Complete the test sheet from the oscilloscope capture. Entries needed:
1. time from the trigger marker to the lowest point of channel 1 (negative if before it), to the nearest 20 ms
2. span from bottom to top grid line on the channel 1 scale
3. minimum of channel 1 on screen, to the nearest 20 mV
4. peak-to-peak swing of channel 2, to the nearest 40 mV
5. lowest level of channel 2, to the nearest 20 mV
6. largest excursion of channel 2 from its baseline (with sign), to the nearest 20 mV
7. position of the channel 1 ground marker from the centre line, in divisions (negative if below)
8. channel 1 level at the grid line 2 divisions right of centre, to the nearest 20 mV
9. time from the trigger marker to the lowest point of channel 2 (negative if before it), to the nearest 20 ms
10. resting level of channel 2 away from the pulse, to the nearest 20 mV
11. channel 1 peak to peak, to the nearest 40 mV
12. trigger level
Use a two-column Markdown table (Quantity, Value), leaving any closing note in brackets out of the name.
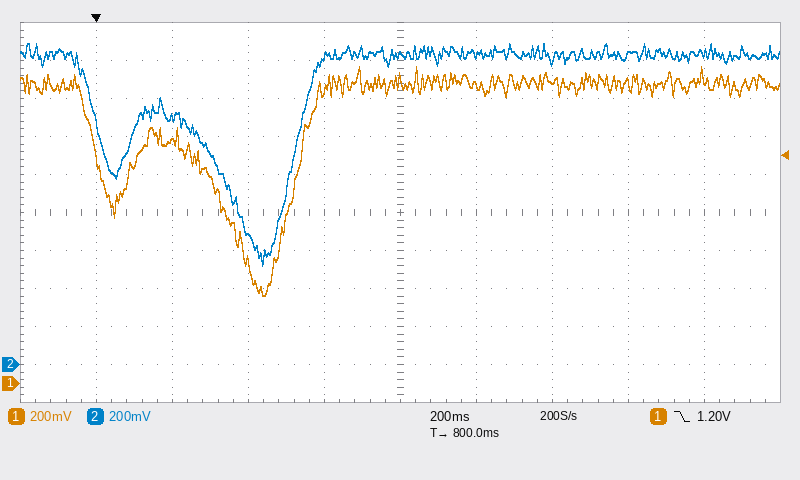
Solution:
| Quantity | Value |
|---|---|
| time from the trigger marker to the lowest point of channel 1 (negative if before it), to the nearest 20 ms | +440 ms |
| span from bottom to top grid line on the channel 1 scale | 2 V |
| minimum of channel 1 on screen, to the nearest 20 mV | 460 mV |
| peak-to-peak swing of channel 2, to the nearest 40 mV | 1.16 V |
| lowest level of channel 2, to the nearest 20 mV | 520 mV |
| largest excursion of channel 2 from its baseline (with sign), to the nearest 20 mV | -1.10 V |
| position of the channel 1 ground marker from the centre line, in divisions | -4.5 div |
| channel 1 level at the grid line 2 divisions right of centre, to the nearest 20 mV | 1.60 V |
| time from the trigger marker to the lowest point of channel 2 (negative if before it), to the nearest 20 ms | +440 ms |
| resting level of channel 2 away from the pulse, to the nearest 20 mV | 1.62 V |
| channel 1 peak to peak, to the nearest 40 mV | 1.20 V |
| trigger level | 1.20 V |
